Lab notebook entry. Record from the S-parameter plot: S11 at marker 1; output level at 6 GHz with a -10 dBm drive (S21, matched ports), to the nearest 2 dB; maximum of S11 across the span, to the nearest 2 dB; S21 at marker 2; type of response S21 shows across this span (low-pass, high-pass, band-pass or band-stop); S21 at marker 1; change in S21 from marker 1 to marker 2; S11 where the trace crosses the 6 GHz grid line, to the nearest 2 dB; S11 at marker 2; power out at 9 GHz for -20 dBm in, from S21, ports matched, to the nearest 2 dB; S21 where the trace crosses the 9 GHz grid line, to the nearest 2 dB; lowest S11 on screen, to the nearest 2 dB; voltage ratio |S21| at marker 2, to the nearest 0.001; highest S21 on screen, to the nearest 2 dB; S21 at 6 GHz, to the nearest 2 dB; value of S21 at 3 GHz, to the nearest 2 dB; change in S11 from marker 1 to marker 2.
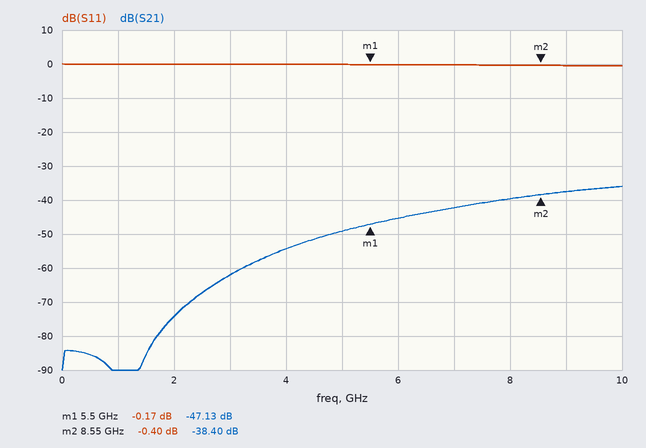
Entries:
-0.17 dB
-56 dBm
0 dB
-38.40 dB
high-pass
-47.13 dB
8.73 dB
0 dB
-0.40 dB
-58 dBm
-38 dB
0 dB
0.012
-36 dB
-46 dB
-62 dB
-0.23 dB
